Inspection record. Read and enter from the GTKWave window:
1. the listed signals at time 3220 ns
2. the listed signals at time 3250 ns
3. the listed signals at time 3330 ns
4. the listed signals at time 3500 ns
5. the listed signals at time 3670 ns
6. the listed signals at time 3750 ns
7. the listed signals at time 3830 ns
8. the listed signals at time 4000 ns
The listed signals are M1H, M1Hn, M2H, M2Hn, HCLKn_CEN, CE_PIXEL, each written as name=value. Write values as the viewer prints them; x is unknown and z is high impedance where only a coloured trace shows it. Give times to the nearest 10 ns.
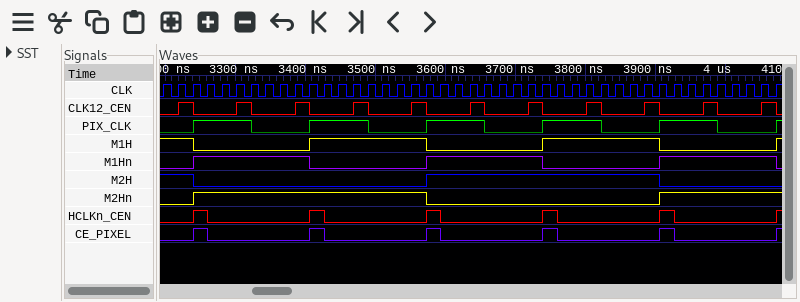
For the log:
M1H=1, M1Hn=0, M2H=1, M2Hn=0, HCLKn_CEN=0, CE_PIXEL=0
M1H=0, M1Hn=1, M2H=0, M2Hn=1, HCLKn_CEN=1, CE_PIXEL=1
M1H=0, M1Hn=1, M2H=0, M2Hn=1, HCLKn_CEN=0, CE_PIXEL=0
M1H=1, M1Hn=0, M2H=0, M2Hn=1, HCLKn_CEN=0, CE_PIXEL=0
M1H=0, M1Hn=1, M2H=1, M2Hn=0, HCLKn_CEN=0, CE_PIXEL=0
M1H=1, M1Hn=0, M2H=1, M2Hn=0, HCLKn_CEN=1, CE_PIXEL=1
M1H=1, M1Hn=0, M2H=1, M2Hn=0, HCLKn_CEN=0, CE_PIXEL=0
M1H=0, M1Hn=1, M2H=0, M2Hn=1, HCLKn_CEN=0, CE_PIXEL=0
